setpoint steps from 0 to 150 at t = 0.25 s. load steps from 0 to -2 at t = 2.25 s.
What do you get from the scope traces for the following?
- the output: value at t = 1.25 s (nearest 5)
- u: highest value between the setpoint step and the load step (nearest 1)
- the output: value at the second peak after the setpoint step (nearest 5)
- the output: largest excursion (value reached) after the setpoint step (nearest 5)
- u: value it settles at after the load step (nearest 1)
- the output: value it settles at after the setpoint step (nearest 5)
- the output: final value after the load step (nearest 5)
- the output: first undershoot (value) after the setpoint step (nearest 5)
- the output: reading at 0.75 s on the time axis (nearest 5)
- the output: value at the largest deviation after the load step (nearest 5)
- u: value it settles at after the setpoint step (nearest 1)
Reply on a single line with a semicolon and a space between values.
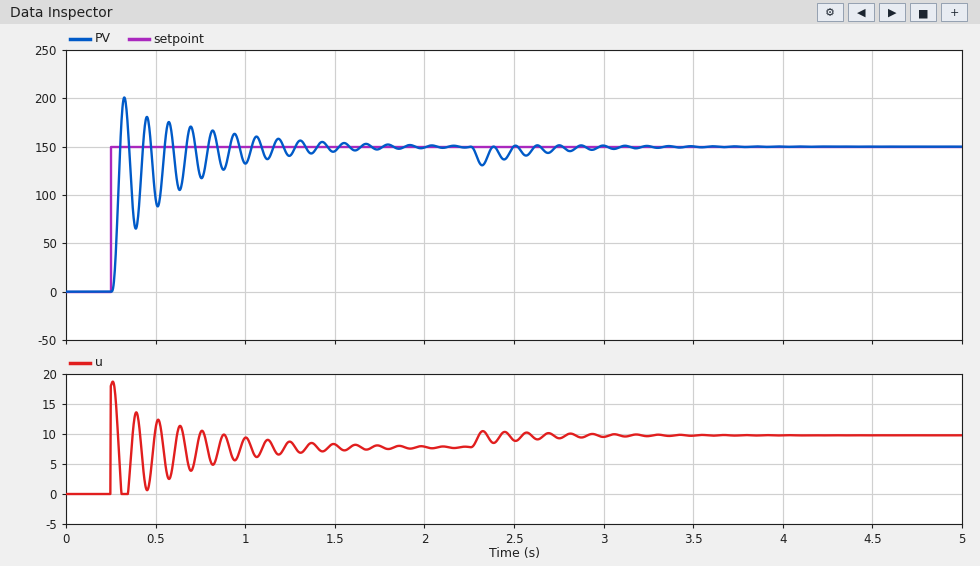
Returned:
140; 19; 180; 200; 10; 150; 150; 65; 120; 130; 8
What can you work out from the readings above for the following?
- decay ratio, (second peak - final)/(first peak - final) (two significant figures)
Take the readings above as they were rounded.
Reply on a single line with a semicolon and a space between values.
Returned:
0.60
